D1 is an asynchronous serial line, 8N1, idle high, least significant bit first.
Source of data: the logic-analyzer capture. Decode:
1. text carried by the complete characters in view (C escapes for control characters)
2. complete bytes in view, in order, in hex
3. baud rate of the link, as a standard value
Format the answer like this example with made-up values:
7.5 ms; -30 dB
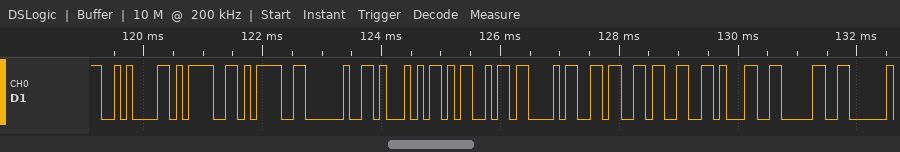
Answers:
"\n== QMC6310"; 0A 3D 3D 20 51 4D 43 36 33 31 30; 9600 baud
